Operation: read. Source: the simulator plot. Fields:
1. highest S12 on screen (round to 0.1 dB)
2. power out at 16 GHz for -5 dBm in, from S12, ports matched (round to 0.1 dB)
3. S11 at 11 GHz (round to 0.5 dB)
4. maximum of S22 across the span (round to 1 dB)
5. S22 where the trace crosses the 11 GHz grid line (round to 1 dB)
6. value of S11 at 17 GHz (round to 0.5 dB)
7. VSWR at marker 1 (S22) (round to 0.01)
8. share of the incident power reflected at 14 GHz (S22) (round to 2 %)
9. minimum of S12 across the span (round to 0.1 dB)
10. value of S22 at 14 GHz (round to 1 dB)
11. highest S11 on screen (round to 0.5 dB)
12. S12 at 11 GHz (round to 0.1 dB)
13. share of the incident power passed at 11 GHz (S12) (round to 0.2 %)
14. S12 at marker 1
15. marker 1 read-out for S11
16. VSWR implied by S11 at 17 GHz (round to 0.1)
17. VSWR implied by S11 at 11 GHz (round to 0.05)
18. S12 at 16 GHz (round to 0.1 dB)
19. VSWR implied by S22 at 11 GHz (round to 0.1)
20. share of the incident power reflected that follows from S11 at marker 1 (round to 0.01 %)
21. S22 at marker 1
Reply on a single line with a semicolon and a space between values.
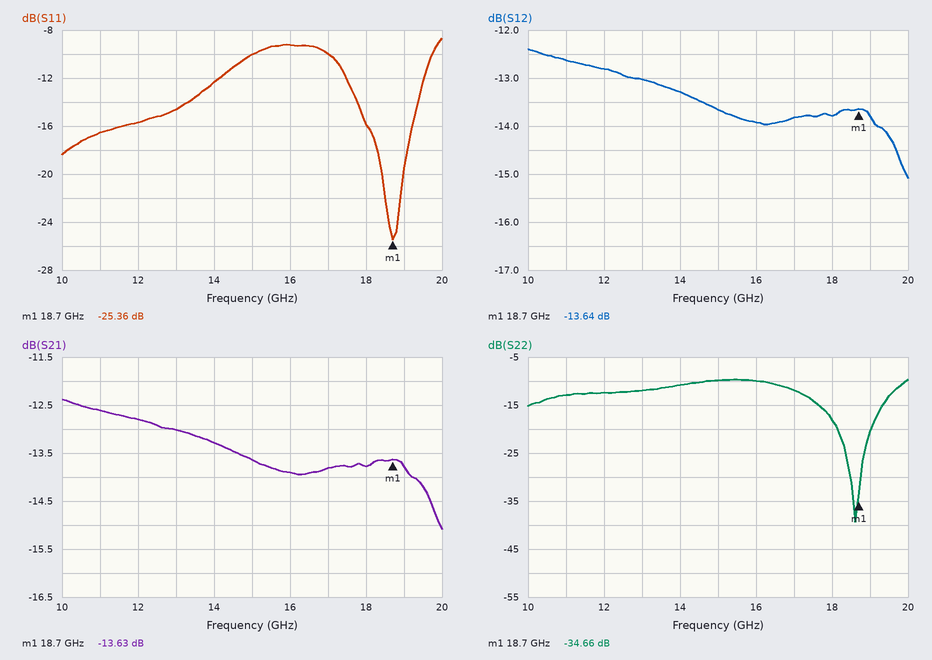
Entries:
-12.4 dB; -18.9 dBm; -16.5 dB; -10 dB; -13 dB; -10.0 dB; 1.04; 8 %; -15.1 dB; -11 dB; -8.5 dB; -12.6 dB; 5.4 %; -13.64 dB; -25.36 dB; 1.9; 1.35; -13.9 dB; 1.6; 0.29 %; -34.66 dB
